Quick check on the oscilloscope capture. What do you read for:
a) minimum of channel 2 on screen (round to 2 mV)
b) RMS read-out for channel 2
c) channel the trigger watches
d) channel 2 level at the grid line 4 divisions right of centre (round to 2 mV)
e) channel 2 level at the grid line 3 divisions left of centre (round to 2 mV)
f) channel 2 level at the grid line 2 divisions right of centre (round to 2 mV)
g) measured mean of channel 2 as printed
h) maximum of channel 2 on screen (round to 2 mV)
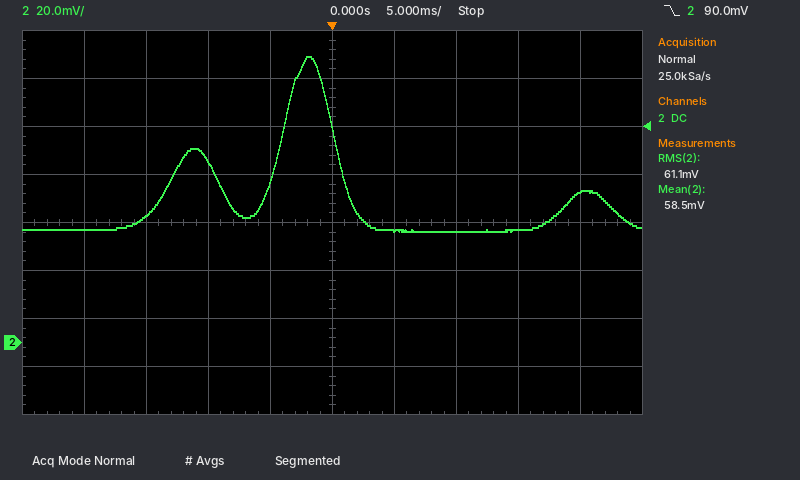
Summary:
46 mV
61.1 mV
channel 2
62 mV
52 mV
46 mV
58.5 mV
120 mV
